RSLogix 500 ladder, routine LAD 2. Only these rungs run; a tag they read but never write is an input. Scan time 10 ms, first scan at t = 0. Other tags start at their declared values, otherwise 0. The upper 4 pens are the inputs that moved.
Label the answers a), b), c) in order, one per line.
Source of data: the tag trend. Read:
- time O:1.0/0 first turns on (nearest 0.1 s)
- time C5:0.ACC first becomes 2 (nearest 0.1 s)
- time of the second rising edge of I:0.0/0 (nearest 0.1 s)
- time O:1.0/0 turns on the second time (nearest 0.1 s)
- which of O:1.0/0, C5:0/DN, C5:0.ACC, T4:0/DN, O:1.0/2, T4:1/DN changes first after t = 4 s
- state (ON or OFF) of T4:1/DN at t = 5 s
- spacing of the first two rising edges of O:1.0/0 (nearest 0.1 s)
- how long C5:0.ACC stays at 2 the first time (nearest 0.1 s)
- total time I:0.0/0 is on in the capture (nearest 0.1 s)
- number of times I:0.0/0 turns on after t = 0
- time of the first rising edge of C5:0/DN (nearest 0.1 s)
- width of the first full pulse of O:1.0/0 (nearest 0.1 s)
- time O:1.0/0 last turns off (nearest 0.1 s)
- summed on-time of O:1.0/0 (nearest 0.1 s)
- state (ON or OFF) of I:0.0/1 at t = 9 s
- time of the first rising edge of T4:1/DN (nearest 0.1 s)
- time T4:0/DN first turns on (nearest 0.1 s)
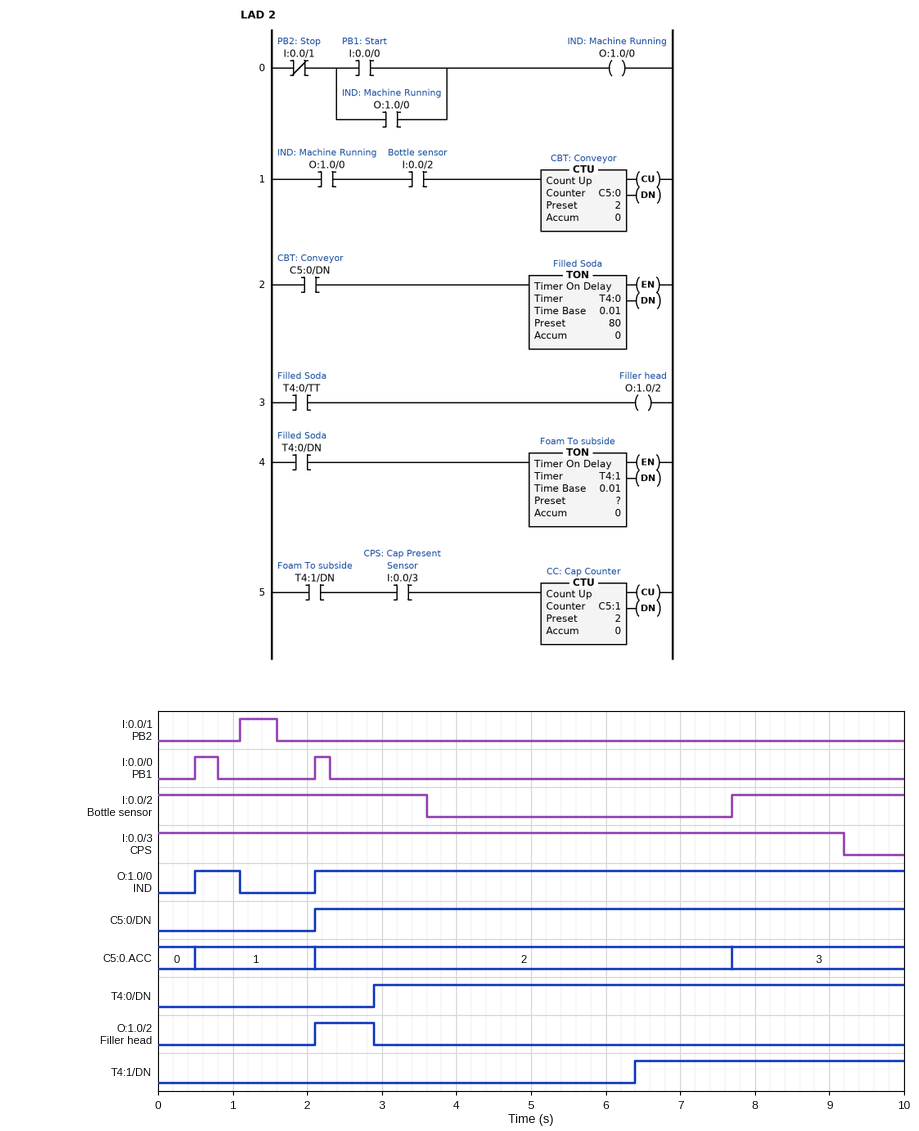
a) 0.5 s
b) 2.1 s
c) 2.1 s
d) 2.1 s
e) T4:1/DN
f) OFF
g) 1.6 s
h) 5.6 s
i) 0.5 s
j) 2
k) 2.1 s
l) 0.6 s
m) 1.1 s
n) 8.5 s
o) OFF
p) 6.4 s
q) 2.9 s
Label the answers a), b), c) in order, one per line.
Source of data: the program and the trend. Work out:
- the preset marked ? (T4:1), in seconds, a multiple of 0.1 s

a) 3.5 s
